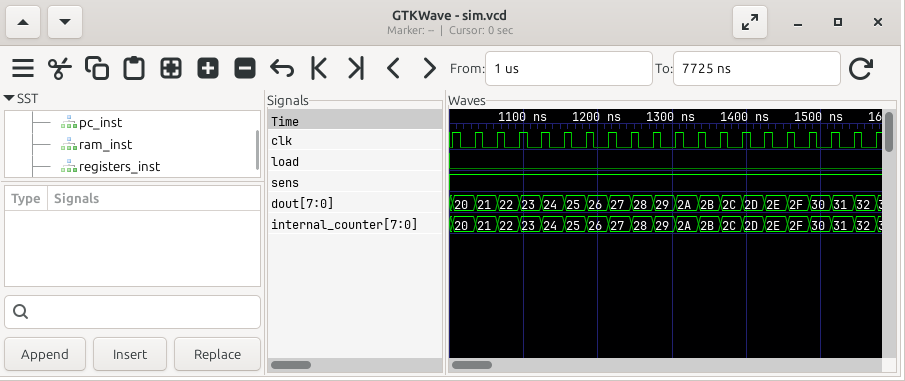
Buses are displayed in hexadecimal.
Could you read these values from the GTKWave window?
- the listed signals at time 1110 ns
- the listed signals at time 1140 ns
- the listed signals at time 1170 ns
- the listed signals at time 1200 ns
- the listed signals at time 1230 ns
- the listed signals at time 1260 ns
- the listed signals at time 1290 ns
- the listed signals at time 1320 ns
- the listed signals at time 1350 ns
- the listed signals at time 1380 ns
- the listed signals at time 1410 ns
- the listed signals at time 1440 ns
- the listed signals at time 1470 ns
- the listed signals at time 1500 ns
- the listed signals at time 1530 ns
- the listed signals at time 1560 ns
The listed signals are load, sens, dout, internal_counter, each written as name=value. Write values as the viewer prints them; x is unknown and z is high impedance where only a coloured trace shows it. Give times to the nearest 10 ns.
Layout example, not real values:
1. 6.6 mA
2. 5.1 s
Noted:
1. load=0, sens=1, dout=23, internal_counter=23
2. load=0, sens=1, dout=24, internal_counter=24
3. load=0, sens=1, dout=25, internal_counter=25
4. load=0, sens=1, dout=26, internal_counter=26
5. load=0, sens=1, dout=27, internal_counter=27
6. load=0, sens=1, dout=28, internal_counter=28
7. load=0, sens=1, dout=29, internal_counter=29
8. load=0, sens=1, dout=2A, internal_counter=2A
9. load=0, sens=1, dout=2B, internal_counter=2B
10. load=0, sens=1, dout=2C, internal_counter=2C
11. load=0, sens=1, dout=2D, internal_counter=2D
12. load=0, sens=1, dout=2E, internal_counter=2E
13. load=0, sens=1, dout=2F, internal_counter=2F
14. load=0, sens=1, dout=30, internal_counter=30
15. load=0, sens=1, dout=31, internal_counter=31
16. load=0, sens=1, dout=32, internal_counter=32
